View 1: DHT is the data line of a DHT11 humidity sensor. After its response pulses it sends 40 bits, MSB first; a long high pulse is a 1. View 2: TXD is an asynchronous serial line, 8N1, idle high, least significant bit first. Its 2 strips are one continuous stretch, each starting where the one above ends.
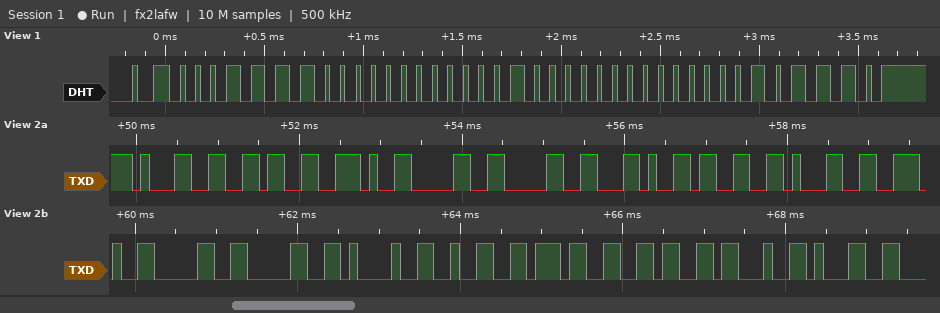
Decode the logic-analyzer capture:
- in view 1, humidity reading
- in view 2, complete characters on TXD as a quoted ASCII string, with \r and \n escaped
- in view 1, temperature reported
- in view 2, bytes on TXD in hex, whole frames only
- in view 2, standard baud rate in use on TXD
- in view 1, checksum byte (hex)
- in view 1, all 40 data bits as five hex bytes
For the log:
30 %
"16.00,31.00!276#1"
16.0 °C
0x31 0x36 0x2E 0x30 0x30 0x2C 0x33 0x31 0x2E 0x30 0x30 0x21 0x32 0x37 0x36 0x23 0x31
9600 baud
0x2E
1E 00 10 00 2E
